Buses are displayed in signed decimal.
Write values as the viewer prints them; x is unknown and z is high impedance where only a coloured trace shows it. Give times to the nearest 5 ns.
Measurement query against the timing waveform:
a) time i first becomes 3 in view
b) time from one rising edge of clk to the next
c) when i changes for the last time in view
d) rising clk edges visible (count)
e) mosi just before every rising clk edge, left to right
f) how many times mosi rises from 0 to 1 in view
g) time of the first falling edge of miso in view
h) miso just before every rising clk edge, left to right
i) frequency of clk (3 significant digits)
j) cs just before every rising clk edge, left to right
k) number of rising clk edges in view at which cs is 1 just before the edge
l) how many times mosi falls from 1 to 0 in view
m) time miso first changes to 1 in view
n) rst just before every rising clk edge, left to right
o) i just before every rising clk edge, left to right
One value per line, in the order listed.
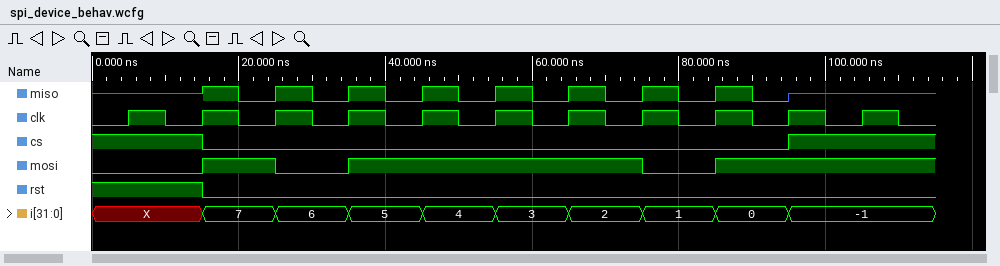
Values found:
55 ns
10 ns
95 ns
11
0 0 1 0 1 1 1 1 0 1 1
3
20 ns
z z 0 0 0 0 0 0 0 0 z
100 MHz
1 1 0 0 0 0 0 0 0 0 1
3
2
15 ns
1 1 0 0 0 0 0 0 0 0 0
X, X, 7, 6, 5, 4, 3, 2, 1, 0, -1
